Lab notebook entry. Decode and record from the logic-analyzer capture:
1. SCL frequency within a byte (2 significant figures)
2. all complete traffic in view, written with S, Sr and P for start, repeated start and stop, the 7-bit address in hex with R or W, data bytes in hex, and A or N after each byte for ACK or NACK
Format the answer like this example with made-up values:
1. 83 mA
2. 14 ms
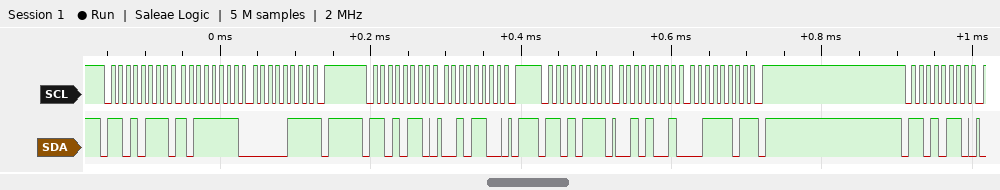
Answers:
1. 100 kHz
2. S 6BR A BF A 07 N P S 6BW A 2C A P S 6BR A 29 A 3D N P S 6BW A
